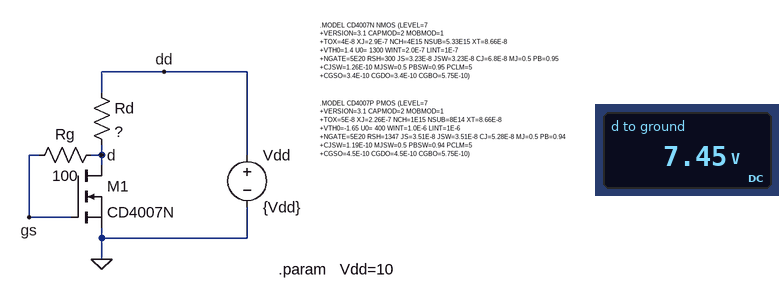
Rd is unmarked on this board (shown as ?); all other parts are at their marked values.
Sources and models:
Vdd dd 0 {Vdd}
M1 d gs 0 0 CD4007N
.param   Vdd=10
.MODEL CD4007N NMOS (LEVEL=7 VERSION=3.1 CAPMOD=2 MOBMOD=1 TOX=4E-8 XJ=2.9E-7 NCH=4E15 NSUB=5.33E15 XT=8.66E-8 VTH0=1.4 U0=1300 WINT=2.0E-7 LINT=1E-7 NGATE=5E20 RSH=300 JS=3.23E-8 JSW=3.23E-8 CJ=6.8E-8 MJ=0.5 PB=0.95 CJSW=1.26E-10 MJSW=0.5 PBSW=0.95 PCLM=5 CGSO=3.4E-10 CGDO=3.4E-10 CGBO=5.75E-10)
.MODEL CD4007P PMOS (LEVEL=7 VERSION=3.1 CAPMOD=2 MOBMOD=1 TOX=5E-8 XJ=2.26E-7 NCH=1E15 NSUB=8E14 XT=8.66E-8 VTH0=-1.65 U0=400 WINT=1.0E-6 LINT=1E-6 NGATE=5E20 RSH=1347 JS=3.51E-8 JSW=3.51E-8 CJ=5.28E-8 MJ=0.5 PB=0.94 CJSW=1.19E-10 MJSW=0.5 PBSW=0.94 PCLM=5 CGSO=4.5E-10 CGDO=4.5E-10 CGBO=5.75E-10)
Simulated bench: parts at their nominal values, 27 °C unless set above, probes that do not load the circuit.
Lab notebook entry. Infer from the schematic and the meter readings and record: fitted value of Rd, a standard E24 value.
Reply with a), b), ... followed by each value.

a) 3.9 kΩ
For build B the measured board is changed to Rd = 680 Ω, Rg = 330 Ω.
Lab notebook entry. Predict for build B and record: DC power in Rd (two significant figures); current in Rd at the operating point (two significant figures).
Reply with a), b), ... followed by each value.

a) 660 µW
b) 990 µA
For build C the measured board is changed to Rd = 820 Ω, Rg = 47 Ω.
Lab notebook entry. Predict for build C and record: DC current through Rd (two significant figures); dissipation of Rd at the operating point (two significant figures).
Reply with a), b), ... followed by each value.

a) 960 µA
b) 760 µW
